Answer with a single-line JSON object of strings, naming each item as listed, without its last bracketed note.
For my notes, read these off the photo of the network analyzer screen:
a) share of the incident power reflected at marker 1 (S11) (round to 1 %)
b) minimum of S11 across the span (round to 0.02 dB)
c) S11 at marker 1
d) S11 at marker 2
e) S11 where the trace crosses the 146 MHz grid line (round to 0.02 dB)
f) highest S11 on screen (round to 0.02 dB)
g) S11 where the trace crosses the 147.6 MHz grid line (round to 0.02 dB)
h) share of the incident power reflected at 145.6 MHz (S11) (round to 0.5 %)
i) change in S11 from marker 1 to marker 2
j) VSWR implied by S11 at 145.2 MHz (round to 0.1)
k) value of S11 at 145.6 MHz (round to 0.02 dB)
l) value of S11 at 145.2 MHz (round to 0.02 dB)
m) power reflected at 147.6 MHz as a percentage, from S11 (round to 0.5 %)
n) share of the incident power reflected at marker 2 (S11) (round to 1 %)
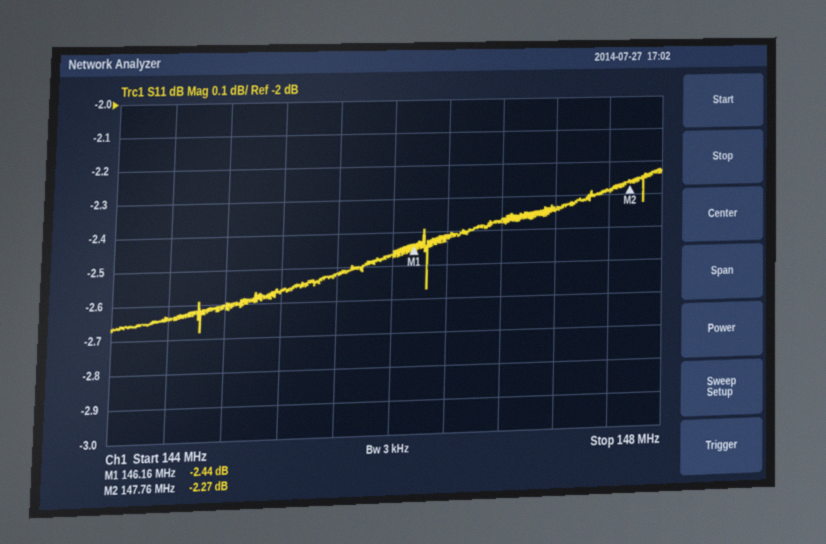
{"share of the incident power reflected at marker 1 (S11)": "57 %", "minimum of S11 across the span": "-2.68 dB", "S11 at marker 1": "-2.44 dB", "S11 at marker 2": "-2.27 dB", "S11 where the trace crosses the 146 MHz grid line": "-2.46 dB", "highest S11 on screen": "-2.22 dB", "S11 where the trace crosses the 147.6 MHz grid line": "-2.28 dB", "share of the incident power reflected at 145.6 MHz (S11)": "56.0 %", "change in S11 from marker 1 to marker 2": "0.17 dB", "VSWR implied by S11 at 145.2 MHz": "6.8", "value of S11 at 145.6 MHz": "-2.52 dB", "value of S11 at 145.2 MHz": "-2.56 dB", "power reflected at 147.6 MHz as a percentage, from S11": "59.0 %", "share of the incident power reflected at marker 2 (S11)": "59 %"}
